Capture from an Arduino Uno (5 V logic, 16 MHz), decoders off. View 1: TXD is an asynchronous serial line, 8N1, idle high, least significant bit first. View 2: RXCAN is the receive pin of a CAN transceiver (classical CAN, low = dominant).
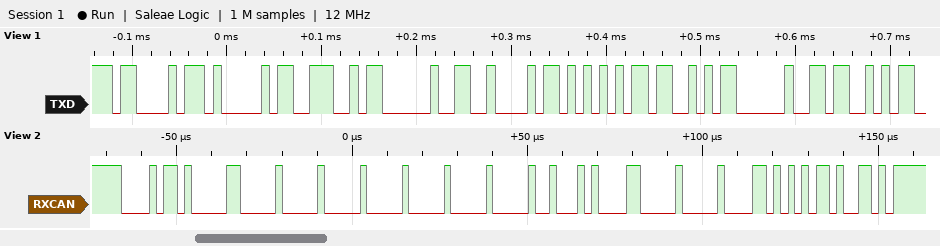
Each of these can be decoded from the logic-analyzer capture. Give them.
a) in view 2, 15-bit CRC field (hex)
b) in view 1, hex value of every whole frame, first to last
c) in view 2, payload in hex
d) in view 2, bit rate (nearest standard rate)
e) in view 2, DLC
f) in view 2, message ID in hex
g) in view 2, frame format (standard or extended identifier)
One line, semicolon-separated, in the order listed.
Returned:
0x55A6; 43 41 4E 20 42 55 53 20 53; 00 00 00 00 22 86 00 06; 500 kbit/s; 8; 0x0B4; standard
